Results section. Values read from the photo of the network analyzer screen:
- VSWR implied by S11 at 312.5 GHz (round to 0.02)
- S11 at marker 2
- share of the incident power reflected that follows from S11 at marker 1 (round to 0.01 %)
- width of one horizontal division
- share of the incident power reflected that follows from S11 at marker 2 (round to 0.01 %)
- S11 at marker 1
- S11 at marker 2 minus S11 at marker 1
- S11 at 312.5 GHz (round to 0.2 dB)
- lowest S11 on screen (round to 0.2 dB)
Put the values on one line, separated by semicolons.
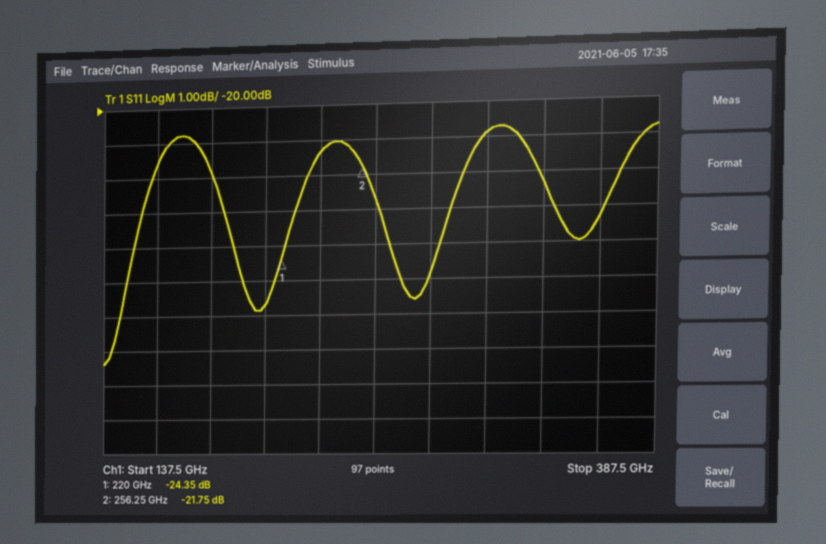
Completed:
1.20; -21.75 dB; 0.37 %; 25 GHz; 0.67 %; -24.35 dB; 2.60 dB; -20.8 dB; -27.4 dB
